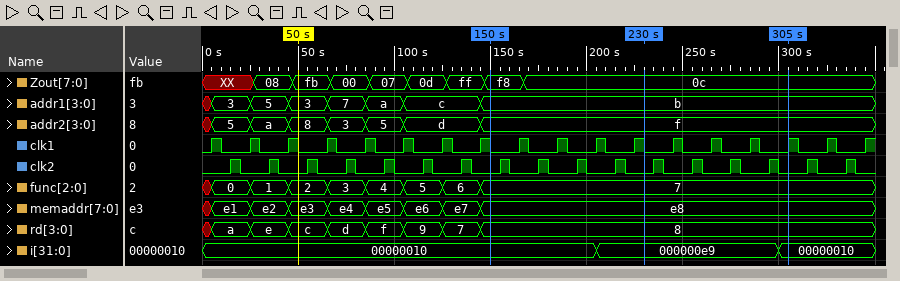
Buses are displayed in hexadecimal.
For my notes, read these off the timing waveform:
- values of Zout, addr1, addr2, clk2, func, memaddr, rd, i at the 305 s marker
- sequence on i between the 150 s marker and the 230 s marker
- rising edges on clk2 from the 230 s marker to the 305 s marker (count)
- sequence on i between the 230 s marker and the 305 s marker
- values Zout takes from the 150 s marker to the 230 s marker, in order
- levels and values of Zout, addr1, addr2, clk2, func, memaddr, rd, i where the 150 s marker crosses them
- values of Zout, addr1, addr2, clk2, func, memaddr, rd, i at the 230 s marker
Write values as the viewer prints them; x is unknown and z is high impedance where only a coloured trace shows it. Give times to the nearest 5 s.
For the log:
Zout=0c, addr1=b, addr2=f, clk2=0, func=7, memaddr=e8, rd=8, i=00000010
00000010, 000000e9
4
000000e9, 00000010
f8, 0c
Zout=f8, addr1=b, addr2=f, clk2=0, func=7, memaddr=e8, rd=8, i=00000010
Zout=0c, addr1=b, addr2=f, clk2=0, func=7, memaddr=e8, rd=8, i=000000e9
